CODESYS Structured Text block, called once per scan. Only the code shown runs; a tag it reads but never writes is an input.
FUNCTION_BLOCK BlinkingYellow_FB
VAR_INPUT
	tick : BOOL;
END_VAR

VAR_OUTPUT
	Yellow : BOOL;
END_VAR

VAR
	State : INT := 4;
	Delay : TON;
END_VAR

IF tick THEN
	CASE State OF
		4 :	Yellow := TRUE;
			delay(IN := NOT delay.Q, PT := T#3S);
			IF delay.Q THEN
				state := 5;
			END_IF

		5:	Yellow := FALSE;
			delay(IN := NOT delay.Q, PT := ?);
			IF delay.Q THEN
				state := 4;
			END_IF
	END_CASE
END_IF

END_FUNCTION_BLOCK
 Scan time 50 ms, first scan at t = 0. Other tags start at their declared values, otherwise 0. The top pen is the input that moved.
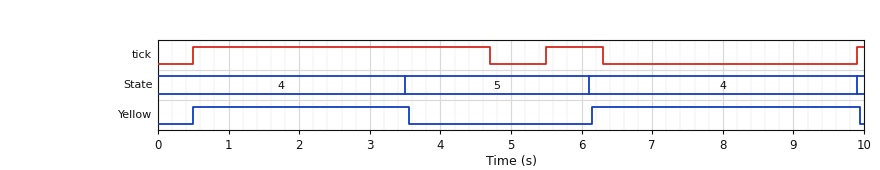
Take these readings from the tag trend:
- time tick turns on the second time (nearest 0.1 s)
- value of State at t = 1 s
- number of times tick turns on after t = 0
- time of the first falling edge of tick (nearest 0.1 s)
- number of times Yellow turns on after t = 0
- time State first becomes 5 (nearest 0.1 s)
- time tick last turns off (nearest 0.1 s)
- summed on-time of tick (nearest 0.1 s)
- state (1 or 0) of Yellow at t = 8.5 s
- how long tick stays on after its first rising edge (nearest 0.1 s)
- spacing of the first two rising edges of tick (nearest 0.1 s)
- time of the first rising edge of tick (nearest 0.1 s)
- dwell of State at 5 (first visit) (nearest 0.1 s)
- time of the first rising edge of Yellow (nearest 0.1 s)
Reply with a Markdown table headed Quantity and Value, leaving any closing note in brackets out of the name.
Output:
| Quantity | Value |
|---|---|
| time tick turns on the second time | 5.5 s |
| value of State at t = 1 s | 4 |
| number of times tick turns on after t = 0 | 3 |
| time of the first falling edge of tick | 4.7 s |
| number of times Yellow turns on after t = 0 | 2 |
| time State first becomes 5 | 3.5 s |
| time tick last turns off | 6.3 s |
| summed on-time of tick | 5.1 s |
| state (1 or 0) of Yellow at t = 8.5 s | 1 |
| how long tick stays on after its first rising edge | 4.2 s |
| spacing of the first two rising edges of tick | 5.0 s |
| time of the first rising edge of tick | 0.5 s |
| dwell of State at 5 (first visit) | 2.6 s |
| time of the first rising edge of Yellow | 0.5 s |
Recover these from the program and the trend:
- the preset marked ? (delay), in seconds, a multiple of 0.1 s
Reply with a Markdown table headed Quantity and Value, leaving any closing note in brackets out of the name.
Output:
| Quantity | Value |
|---|---|
| the preset marked ? (delay), in seconds, a multiple of 0.1 s | 2.5 s |
